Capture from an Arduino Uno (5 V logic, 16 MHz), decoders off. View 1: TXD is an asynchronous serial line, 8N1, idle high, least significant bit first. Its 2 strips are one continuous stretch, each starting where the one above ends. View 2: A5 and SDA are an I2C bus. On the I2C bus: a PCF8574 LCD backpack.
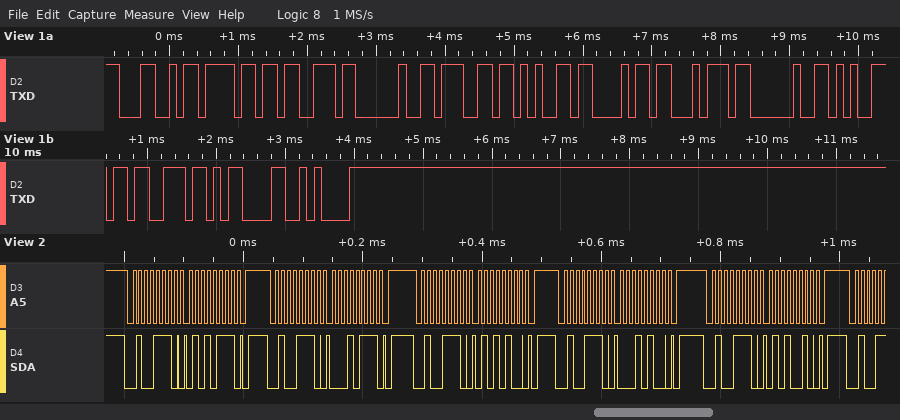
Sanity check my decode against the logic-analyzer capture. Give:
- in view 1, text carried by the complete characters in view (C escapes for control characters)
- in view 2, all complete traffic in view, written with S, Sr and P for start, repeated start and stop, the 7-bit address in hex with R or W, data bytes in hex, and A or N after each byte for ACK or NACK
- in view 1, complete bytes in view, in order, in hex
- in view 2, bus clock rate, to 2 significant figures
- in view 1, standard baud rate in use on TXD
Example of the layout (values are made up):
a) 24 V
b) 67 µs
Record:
a) "Los geht es\r\n"
b) S 27W A 57 A P S 27W A 17 A P S 27W A 54 A P S 27W A 14 A P S 27W A 52 A P
c) 0x4C 0x6F 0x73 0x20 0x67 0x65 0x68 0x74 0x20 0x65 0x73 0x0D 0x0A
d) 100 kHz
e) 9600 baud
